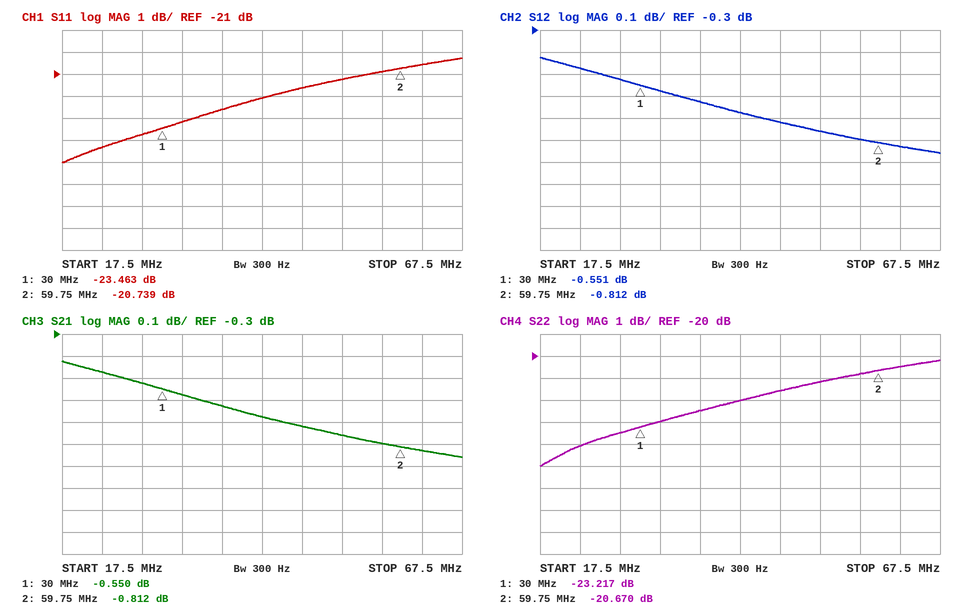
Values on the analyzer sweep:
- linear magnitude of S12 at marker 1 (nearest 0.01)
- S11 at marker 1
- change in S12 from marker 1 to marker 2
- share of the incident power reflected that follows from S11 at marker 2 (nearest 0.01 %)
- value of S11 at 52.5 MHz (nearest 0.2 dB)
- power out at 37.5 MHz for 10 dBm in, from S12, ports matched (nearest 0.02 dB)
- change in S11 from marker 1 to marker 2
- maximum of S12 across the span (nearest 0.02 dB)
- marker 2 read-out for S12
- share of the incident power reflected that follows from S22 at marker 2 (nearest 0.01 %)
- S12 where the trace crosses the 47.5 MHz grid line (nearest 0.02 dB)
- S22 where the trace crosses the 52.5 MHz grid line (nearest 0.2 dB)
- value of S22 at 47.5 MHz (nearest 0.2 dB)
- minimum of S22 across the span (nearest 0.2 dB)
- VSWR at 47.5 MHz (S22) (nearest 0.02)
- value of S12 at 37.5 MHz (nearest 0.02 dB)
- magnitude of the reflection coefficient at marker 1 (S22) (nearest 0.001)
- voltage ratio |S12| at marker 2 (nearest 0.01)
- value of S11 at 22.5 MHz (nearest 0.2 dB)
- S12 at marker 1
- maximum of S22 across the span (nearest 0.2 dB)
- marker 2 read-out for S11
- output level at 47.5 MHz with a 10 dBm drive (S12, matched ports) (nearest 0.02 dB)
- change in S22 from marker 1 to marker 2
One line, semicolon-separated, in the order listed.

0.94; -23.463 dB; -0.261 dB; 0.84 %; -21.2 dB; 9.38 dBm; 2.724 dB; -0.42 dB; -0.812 dB; 0.86 %; -0.72 dB; -21.2 dB; -21.6 dB; -25.0 dB; 1.18; -0.62 dB; 0.069; 0.91; -24.4 dB; -0.551 dB; -20.2 dB; -20.739 dB; 9.28 dBm; 2.547 dB
